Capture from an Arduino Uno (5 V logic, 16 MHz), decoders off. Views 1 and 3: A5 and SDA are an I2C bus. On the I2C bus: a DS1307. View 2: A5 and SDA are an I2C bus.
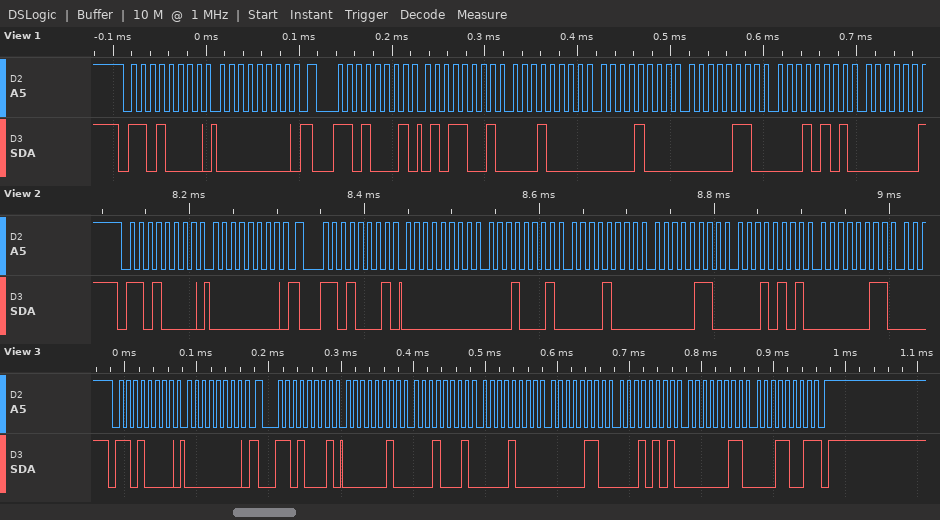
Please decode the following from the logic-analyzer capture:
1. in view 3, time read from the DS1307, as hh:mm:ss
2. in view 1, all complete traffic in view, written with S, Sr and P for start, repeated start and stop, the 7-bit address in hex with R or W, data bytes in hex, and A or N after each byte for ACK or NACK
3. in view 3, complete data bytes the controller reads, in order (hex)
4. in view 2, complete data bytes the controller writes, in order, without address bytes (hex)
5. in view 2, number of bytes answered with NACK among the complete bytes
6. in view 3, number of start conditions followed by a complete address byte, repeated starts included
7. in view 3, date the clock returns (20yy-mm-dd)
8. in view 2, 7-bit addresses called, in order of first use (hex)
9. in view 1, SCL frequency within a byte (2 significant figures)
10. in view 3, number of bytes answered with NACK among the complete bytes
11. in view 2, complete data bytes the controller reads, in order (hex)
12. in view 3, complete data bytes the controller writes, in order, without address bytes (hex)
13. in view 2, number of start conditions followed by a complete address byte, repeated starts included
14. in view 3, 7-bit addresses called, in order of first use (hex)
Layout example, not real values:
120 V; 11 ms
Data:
08:11:02; S 68W A 00 A Sr 68R A 59 A 10 A 08 A 06 A 15 A; 02 11 08 06 15 03 19; 00; 0; 2; 2019-03-15; 0x68; 100 kHz; 1; 00 11 08 06 15 03; 00; 2; 0x68
